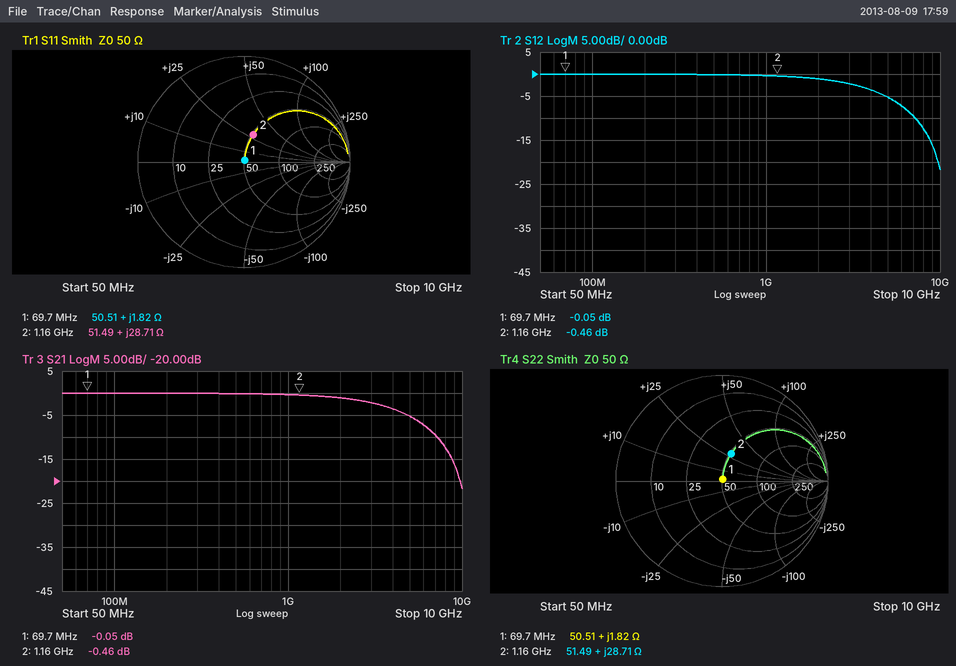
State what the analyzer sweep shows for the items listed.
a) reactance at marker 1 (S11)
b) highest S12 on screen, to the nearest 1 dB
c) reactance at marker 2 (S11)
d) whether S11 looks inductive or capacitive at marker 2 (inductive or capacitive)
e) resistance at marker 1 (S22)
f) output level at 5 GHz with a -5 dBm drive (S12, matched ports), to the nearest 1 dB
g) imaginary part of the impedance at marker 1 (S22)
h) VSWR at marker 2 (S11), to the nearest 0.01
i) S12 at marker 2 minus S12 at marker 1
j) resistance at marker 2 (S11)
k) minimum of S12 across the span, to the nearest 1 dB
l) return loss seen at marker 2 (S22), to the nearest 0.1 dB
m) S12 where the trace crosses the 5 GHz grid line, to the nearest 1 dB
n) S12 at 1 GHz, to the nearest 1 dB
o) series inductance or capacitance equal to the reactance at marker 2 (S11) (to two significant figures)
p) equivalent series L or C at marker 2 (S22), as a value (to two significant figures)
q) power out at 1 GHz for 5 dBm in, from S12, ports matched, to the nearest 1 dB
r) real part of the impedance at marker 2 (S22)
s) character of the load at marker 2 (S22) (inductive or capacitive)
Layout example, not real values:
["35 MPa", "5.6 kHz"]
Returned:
["+1.82 Ω", "0 dB", "+28.71 Ω", "inductive", "50.51 Ω", "-10 dBm", "+1.82 Ω", "1.75", "-0.41 dB", "51.49 Ω", "-22 dB", "11.3 dB", "-5 dB", "0 dB", "3.9 nH", "3.9 nH", "5 dBm", "51.49 Ω", "inductive"]
